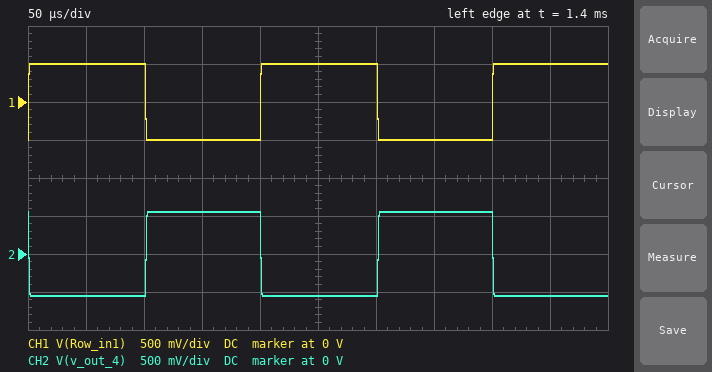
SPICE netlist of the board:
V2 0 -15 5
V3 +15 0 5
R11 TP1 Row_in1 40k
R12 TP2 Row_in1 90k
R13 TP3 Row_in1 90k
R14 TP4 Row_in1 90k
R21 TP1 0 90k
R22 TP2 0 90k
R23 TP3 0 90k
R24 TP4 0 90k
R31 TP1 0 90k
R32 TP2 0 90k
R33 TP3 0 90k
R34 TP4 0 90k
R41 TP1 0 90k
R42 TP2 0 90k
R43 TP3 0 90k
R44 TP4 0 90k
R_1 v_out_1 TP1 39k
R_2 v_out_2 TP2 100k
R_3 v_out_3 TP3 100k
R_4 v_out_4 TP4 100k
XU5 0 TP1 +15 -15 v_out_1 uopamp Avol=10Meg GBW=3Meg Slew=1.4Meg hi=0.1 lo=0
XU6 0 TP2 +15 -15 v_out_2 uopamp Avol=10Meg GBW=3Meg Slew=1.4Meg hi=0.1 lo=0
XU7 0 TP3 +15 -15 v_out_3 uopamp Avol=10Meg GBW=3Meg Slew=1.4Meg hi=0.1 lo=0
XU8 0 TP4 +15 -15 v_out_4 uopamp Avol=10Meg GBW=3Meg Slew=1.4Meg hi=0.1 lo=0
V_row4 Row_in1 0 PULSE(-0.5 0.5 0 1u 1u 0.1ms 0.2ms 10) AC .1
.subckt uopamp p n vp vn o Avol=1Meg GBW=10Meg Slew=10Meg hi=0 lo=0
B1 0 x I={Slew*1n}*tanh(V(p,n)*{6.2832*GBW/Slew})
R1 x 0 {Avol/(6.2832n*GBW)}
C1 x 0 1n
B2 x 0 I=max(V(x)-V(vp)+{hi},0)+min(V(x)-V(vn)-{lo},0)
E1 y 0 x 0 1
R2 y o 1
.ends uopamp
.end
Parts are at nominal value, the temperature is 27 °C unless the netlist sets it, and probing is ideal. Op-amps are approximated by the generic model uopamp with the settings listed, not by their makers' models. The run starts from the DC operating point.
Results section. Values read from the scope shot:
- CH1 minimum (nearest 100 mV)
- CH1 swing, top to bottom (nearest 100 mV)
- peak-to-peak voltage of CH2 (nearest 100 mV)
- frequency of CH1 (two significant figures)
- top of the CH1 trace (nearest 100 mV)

-500 mV
1.0 V
1.1 V
5.0 kHz
500 mV
